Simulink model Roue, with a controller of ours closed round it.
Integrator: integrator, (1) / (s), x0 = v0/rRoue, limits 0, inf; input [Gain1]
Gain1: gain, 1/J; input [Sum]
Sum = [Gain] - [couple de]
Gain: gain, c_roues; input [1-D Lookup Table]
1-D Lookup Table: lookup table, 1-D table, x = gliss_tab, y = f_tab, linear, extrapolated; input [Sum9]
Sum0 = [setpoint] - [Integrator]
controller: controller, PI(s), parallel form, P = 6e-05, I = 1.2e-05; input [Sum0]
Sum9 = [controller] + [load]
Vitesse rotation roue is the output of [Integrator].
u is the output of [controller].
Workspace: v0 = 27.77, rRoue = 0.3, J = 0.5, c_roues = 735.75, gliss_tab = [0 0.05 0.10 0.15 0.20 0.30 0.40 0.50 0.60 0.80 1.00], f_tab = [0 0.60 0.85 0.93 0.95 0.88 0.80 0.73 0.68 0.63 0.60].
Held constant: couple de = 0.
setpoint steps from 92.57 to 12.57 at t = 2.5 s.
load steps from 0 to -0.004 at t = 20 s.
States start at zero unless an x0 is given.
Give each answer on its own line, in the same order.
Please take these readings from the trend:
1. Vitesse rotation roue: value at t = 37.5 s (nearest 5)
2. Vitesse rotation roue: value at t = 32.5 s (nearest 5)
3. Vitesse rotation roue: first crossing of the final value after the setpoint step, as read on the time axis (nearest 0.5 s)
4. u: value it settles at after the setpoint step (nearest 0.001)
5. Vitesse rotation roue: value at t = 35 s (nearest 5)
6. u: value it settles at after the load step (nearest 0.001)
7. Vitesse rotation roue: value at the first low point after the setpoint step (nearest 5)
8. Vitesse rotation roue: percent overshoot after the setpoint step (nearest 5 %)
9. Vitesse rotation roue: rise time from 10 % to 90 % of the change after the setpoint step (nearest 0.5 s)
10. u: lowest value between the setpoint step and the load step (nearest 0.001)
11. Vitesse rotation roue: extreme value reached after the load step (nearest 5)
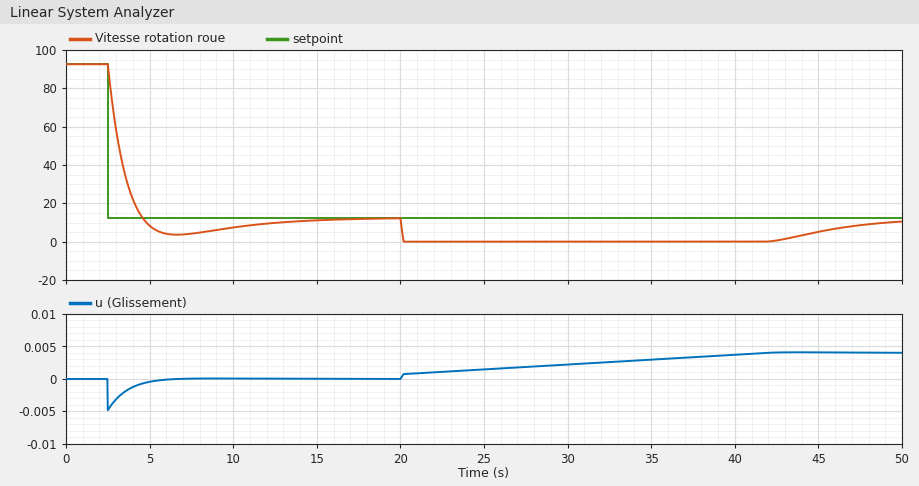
0
0
4.5 s
0.000
0
0.004
5
10 %
1.5 s
-0.005
0
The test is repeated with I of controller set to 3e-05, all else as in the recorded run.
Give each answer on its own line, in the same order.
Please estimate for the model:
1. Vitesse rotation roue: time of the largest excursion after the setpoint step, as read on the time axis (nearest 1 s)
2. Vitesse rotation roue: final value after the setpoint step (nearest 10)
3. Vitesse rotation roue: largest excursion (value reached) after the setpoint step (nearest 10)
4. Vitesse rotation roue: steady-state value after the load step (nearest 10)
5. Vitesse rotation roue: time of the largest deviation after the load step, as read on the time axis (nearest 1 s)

5 s
10
0
10
20 s
